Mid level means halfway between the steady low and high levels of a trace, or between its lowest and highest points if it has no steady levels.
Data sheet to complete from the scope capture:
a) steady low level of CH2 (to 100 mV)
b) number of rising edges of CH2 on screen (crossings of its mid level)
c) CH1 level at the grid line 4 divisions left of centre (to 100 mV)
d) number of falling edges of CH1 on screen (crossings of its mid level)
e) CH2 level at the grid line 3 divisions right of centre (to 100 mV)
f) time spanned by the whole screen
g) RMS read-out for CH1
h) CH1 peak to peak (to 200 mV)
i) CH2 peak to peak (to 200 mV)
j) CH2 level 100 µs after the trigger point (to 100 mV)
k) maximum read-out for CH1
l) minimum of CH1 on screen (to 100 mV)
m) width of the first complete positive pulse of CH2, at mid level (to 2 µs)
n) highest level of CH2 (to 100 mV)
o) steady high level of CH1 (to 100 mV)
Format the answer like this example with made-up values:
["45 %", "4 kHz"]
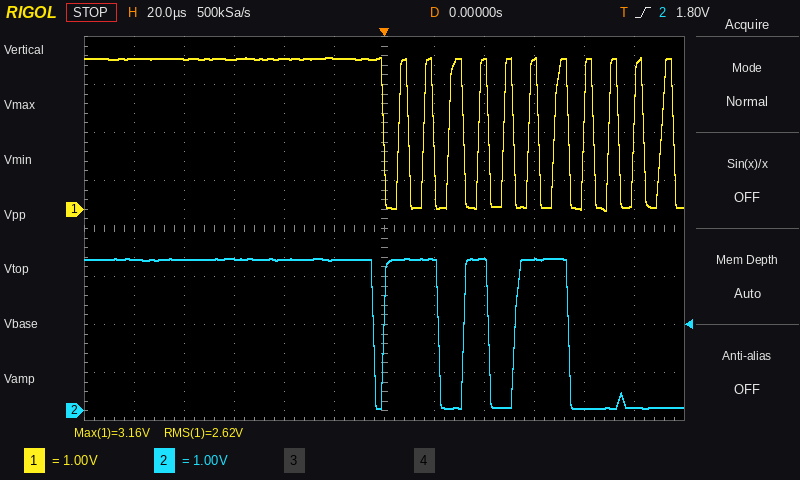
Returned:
["100 mV", "3", "3.1 V", "12", "3.2 V", "240 µs", "2.62 V", "3.2 V", "3.2 V", "100 mV", "3.16 V", "0.0 V", "22 µs", "3.2 V", "3.1 V"]
